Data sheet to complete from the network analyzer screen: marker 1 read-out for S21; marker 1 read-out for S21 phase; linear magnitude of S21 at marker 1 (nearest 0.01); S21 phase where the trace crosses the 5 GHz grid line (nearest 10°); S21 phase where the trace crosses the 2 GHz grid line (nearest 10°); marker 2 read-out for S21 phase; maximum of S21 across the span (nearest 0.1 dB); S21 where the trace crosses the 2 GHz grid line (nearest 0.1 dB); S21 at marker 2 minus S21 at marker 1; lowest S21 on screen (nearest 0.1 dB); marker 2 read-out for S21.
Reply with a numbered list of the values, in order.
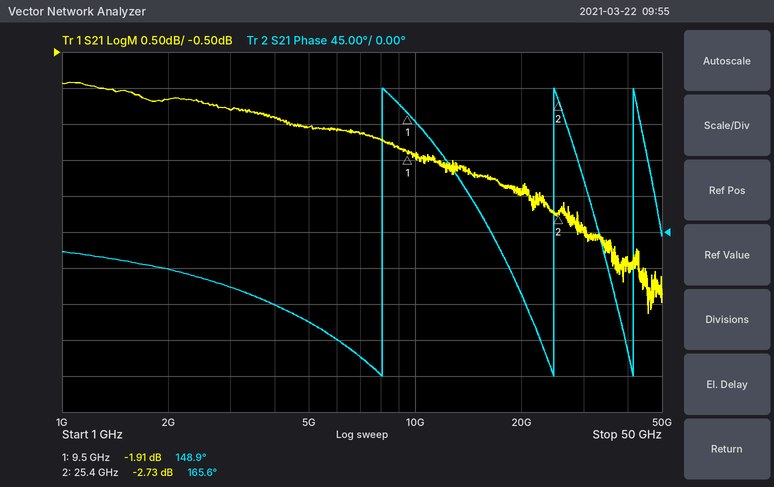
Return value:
1. -1.91 dB
2. 148.9°
3. 0.80
4. -110°
5. -50°
6. 165.6°
7. -0.9 dB
8. -1.2 dB
9. -0.82 dB
10. -4.1 dB
11. -2.73 dB
